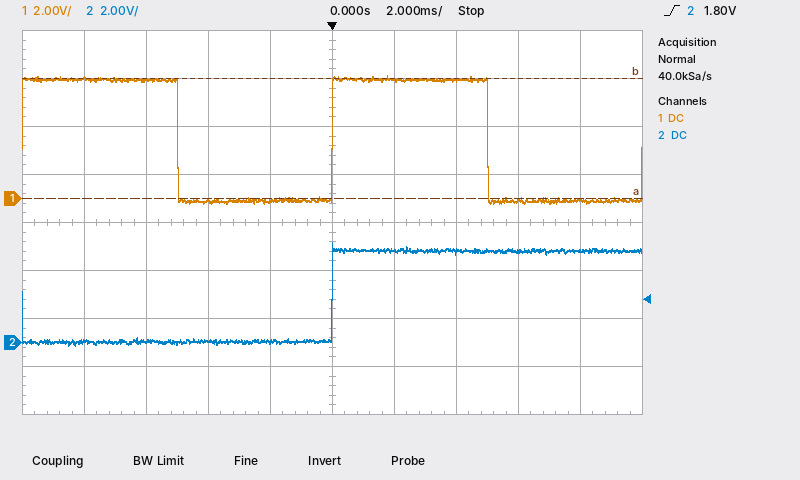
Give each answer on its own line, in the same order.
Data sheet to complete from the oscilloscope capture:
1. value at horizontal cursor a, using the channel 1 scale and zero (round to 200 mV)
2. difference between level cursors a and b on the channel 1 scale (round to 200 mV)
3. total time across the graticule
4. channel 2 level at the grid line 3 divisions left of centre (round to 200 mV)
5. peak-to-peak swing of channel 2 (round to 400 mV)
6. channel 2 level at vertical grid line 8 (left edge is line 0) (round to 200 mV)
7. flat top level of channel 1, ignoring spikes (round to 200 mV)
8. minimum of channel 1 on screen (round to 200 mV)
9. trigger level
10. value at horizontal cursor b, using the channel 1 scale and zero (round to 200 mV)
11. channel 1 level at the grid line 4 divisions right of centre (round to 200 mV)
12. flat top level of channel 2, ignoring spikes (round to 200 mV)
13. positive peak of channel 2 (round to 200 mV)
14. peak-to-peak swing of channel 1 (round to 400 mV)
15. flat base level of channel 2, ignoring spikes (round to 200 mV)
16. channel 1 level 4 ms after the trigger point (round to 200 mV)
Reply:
0.0 V
5.0 V
20 ms
0.0 V
4.4 V
3.8 V
5.0 V
-200 mV
1.80 V
5.0 V
0.0 V
3.8 V
4.2 V
5.2 V
0.0 V
5.0 V
